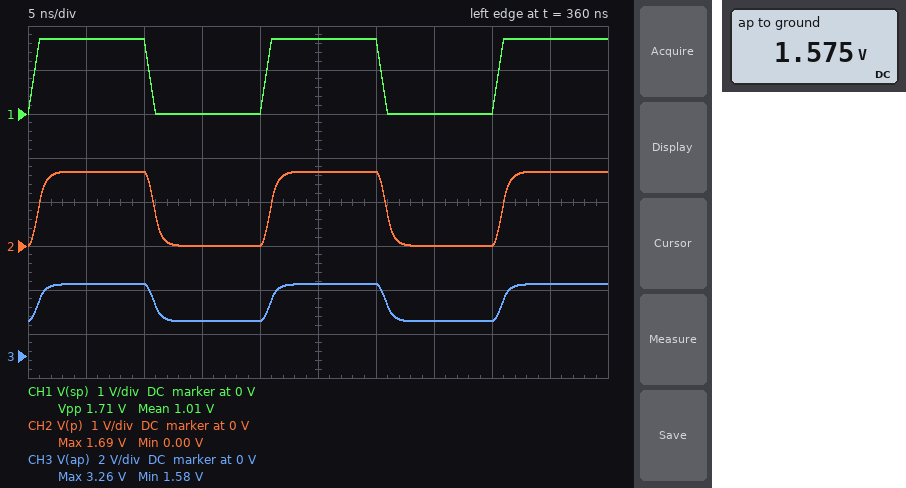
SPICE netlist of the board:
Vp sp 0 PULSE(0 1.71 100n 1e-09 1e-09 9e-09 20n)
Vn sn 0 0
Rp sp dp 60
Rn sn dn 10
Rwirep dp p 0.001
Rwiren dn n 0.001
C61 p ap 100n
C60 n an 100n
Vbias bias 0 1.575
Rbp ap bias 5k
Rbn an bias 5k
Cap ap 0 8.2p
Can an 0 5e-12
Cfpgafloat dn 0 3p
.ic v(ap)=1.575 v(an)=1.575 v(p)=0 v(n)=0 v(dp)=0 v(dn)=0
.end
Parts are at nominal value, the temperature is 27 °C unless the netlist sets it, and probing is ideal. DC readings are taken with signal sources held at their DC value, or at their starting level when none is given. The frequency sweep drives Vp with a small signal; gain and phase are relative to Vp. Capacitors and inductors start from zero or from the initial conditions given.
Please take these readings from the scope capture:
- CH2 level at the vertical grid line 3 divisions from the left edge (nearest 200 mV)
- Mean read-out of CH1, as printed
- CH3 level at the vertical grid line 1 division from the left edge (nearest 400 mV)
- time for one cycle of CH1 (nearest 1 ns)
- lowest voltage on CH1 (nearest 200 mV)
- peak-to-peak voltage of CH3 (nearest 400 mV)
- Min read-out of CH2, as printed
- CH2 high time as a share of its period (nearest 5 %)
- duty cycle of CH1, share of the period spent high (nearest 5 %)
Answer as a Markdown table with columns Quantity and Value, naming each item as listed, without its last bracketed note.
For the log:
| Quantity | Value |
|---|---|
| CH2 level at the vertical grid line 3 divisions from the left edge | 0 V |
| Mean read-out of CH1, as printed | 1.01 V |
| CH3 level at the vertical grid line 1 division from the left edge | 3.2 V |
| time for one cycle of CH1 | 20 ns |
| lowest voltage on CH1 | 0 V |
| peak-to-peak voltage of CH3 | 1.6 V |
| Min read-out of CH2, as printed | 0.00 V |
| CH2 high time as a share of its period | 50 % |
| duty cycle of CH1, share of the period spent high | 50 % |
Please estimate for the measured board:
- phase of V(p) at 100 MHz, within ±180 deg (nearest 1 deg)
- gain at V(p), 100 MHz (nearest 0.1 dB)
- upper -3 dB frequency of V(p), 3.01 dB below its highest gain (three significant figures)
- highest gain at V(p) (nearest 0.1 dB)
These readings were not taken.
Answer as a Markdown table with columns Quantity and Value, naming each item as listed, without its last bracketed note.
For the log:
| Quantity | Value |
|---|---|
| phase of V(p) at 100 MHz, within ±180 deg | -17 deg |
| gain at V(p), 100 MHz | -0.5 dB |
| upper -3 dB frequency of V(p), 3.01 dB below its highest gain | 327 MHz |
| highest gain at V(p) | -0.1 dB |
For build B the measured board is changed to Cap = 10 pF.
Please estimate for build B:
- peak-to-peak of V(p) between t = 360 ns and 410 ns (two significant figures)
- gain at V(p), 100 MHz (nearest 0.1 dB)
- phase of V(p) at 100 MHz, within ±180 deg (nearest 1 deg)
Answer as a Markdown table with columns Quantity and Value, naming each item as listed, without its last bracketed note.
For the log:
| Quantity | Value |
|---|---|
| peak-to-peak of V(p) between t = 360 ns and 410 ns | 1.7 V |
| gain at V(p), 100 MHz | -0.7 dB |
| phase of V(p) at 100 MHz, within ±180 deg | -20 deg |
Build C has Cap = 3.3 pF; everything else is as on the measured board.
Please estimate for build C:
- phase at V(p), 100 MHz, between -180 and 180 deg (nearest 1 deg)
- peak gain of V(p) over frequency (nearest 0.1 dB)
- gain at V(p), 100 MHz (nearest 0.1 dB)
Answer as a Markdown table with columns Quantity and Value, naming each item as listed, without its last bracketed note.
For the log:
| Quantity | Value |
|---|---|
| phase at V(p), 100 MHz, between -180 and 180 deg | -7 deg |
| peak gain of V(p) over frequency | -0.1 dB |
| gain at V(p), 100 MHz | -0.2 dB |
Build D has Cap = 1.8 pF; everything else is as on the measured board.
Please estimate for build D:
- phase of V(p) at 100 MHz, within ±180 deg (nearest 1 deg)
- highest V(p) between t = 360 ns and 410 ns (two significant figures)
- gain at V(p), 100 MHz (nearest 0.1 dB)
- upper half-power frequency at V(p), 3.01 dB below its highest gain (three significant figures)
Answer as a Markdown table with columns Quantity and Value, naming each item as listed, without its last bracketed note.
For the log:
| Quantity | Value |
|---|---|
| phase of V(p) at 100 MHz, within ±180 deg | -4 deg |
| highest V(p) between t = 360 ns and 410 ns | 1.7 V |
| gain at V(p), 100 MHz | -0.1 dB |
| upper half-power frequency at V(p), 3.01 dB below its highest gain | 1.49 GHz |
